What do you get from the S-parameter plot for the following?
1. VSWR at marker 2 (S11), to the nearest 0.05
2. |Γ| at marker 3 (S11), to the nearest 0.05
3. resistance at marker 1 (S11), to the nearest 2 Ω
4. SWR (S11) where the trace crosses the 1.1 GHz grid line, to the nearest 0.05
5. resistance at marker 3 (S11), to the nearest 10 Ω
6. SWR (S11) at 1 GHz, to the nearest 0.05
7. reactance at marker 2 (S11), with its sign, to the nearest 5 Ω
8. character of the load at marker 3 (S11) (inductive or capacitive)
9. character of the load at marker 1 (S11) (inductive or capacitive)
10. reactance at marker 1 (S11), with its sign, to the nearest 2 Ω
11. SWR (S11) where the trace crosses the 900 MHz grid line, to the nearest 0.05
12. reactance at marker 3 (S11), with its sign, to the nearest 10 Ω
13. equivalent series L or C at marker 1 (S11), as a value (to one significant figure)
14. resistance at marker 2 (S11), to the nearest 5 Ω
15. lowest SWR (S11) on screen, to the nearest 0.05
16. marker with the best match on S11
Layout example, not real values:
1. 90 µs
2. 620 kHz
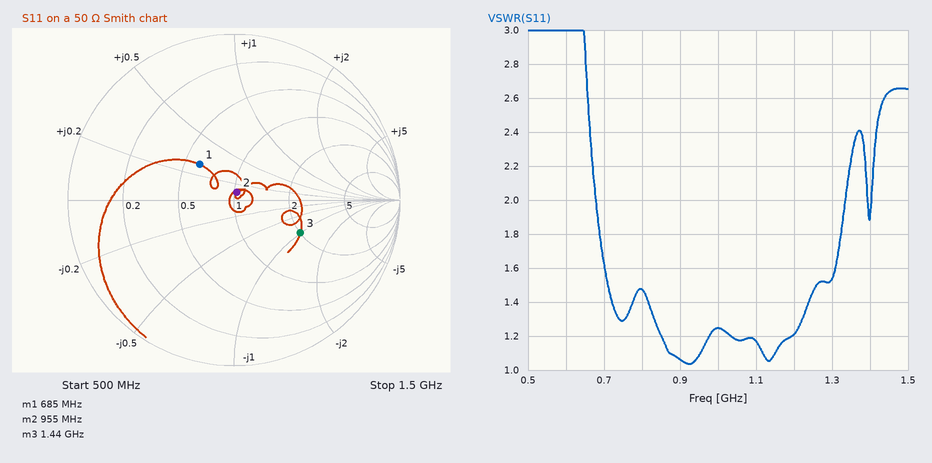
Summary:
1. 1.10
2. 0.45
3. 30 Ω
4. 1.15
5. 100 Ω
6. 1.25
7. +5 Ω
8. capacitive
9. inductive
10. +14 Ω
11. 1.05
12. -50 Ω
13. 3 nH
14. 50 Ω
15. 1.05
16. marker 2
